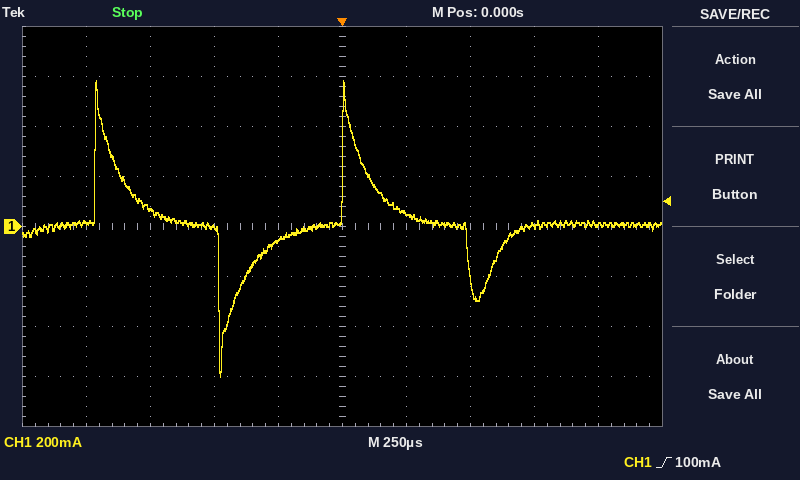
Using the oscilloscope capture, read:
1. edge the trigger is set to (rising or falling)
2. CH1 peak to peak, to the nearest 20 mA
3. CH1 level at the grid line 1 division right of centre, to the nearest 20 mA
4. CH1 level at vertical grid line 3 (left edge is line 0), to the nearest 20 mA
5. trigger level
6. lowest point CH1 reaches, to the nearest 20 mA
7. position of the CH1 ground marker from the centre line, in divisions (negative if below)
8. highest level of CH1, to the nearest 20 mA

rising
1.18 A
60 mA
0 mA
100 mA
-600 mA
0.0 div
580 mA
